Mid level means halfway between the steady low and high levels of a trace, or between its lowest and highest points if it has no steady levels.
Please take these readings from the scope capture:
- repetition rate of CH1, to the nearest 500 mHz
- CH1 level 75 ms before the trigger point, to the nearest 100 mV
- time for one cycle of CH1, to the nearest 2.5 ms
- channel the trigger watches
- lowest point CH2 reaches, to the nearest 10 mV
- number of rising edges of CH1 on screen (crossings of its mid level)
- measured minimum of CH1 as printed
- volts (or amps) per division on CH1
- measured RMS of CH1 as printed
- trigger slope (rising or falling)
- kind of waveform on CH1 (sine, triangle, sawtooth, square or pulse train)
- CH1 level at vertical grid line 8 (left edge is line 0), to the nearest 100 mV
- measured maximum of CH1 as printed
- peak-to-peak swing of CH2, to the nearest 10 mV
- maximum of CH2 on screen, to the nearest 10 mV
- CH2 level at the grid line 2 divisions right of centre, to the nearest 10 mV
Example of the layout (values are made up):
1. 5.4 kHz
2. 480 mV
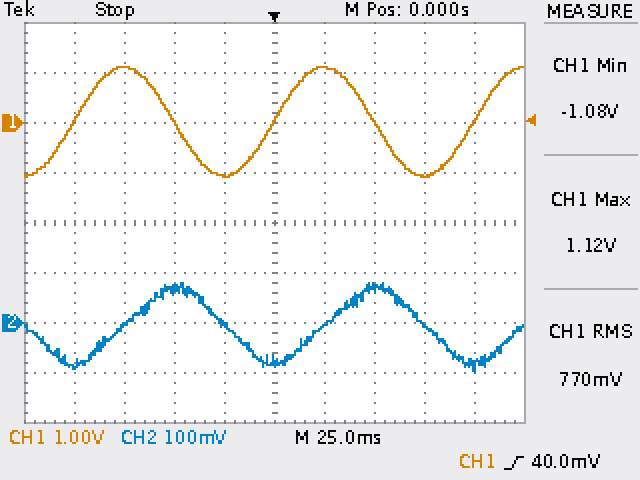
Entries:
1. 10.0 Hz
2. 1.1 V
3. 100.0 ms
4. CH1
5. -100 mV
6. 3
7. -1.08 V
8. 1 V
9. 770 mV
10. rising
11. sine
12. -1.1 V
13. 1.12 V
14. 180 mV
15. 80 mV
16. 70 mV
